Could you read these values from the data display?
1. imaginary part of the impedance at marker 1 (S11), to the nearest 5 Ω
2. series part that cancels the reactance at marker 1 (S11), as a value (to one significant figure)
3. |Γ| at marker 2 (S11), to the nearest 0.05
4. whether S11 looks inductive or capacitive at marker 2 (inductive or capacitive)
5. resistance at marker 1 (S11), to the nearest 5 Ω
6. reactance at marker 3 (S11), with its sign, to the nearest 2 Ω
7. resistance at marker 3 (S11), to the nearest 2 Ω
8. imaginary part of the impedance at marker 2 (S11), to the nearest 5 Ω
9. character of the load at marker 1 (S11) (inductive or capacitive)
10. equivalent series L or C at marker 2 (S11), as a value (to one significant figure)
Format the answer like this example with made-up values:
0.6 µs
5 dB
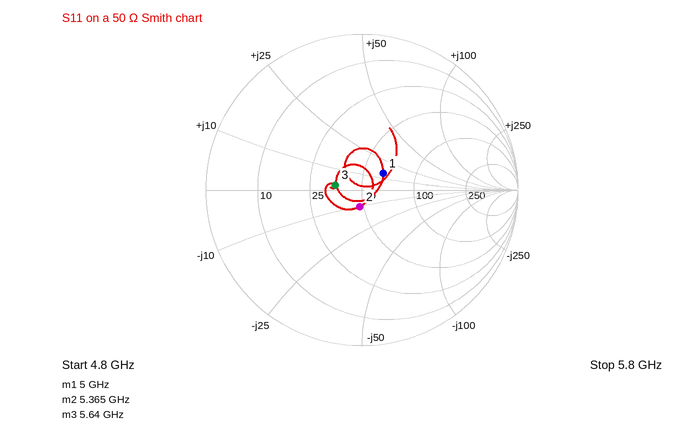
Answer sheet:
+15 Ω
2 pF
0.10
capacitive
65 Ω
+2 Ω
36 Ω
-10 Ω
inductive
3 pF
